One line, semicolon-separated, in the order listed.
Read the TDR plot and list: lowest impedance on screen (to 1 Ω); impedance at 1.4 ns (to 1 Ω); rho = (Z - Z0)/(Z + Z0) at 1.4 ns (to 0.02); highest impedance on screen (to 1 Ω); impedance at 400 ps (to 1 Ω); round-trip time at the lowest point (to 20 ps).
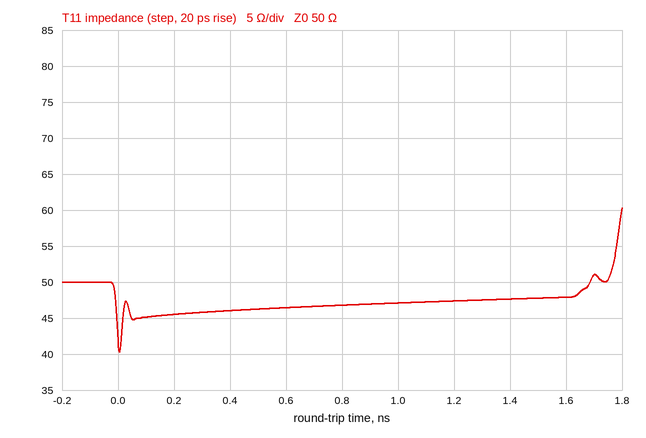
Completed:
40 Ω; 48 Ω; -0.02; 60 Ω; 46 Ω; 0 ps
